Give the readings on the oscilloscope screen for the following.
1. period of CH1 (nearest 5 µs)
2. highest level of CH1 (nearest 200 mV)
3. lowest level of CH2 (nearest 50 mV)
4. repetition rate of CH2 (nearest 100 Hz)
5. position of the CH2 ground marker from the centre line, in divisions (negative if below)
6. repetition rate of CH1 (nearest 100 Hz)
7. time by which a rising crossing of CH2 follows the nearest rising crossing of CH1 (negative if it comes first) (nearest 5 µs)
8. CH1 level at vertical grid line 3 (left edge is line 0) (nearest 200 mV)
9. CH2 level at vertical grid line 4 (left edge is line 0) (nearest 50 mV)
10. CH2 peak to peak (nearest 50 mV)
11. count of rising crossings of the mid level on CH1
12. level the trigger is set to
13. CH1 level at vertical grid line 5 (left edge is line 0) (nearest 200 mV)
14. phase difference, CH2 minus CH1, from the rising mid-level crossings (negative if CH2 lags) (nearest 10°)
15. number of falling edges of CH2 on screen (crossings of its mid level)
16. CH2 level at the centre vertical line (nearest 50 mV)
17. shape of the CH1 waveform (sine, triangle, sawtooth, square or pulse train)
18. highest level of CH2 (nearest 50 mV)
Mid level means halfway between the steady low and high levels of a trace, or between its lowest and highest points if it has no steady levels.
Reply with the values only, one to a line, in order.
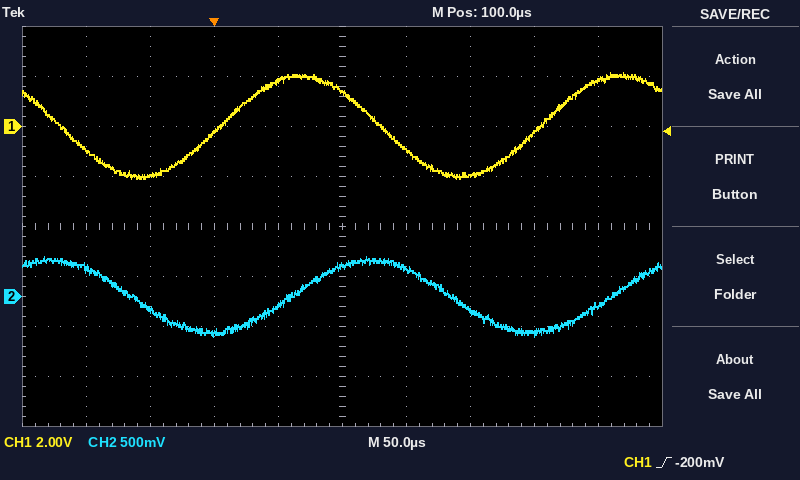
250 µs
2.2 V
-400 mV
4.0 kHz
-1.4 div
4.0 kHz
+55 µs
-200 mV
-100 mV
800 mV
2
-200 mV
1.4 V
-80°
2
300 mV
sine
400 mV
